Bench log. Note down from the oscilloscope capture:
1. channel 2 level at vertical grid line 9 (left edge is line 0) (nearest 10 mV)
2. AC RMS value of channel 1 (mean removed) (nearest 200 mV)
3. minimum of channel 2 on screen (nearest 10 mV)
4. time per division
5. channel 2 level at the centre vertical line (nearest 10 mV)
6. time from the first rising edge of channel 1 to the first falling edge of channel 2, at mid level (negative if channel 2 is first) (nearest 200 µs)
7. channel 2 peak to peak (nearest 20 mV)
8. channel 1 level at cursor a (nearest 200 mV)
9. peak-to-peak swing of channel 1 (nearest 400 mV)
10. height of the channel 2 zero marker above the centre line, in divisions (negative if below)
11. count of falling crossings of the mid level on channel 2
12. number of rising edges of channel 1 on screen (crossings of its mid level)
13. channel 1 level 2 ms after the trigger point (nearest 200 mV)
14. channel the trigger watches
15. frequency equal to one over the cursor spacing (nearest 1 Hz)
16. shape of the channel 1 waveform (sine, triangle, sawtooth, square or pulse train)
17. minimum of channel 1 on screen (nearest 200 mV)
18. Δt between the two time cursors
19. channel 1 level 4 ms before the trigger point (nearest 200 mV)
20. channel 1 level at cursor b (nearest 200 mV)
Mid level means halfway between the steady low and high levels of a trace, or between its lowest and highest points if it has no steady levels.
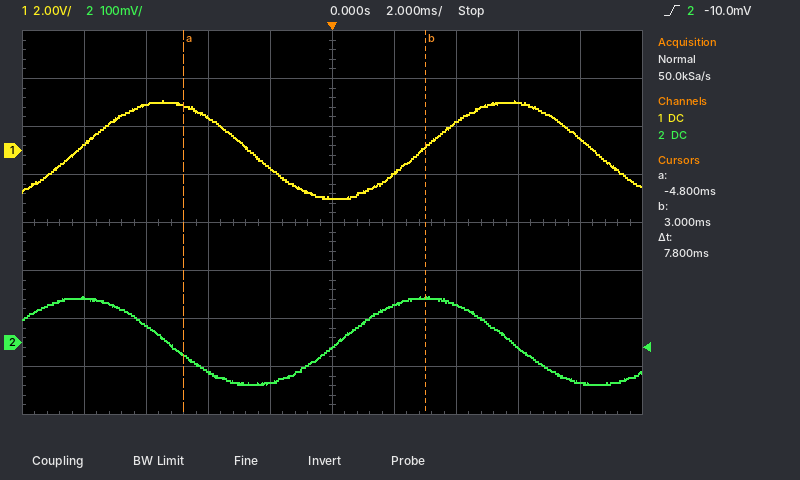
-80 mV
1.4 V
-90 mV
2 ms
-10 mV
+2.8 ms
180 mV
1.8 V
4.0 V
-2.5 div
2
2
-1.0 V
channel 2
128 Hz
sine
-2.0 V
7.8 ms
1.4 V
200 mV
